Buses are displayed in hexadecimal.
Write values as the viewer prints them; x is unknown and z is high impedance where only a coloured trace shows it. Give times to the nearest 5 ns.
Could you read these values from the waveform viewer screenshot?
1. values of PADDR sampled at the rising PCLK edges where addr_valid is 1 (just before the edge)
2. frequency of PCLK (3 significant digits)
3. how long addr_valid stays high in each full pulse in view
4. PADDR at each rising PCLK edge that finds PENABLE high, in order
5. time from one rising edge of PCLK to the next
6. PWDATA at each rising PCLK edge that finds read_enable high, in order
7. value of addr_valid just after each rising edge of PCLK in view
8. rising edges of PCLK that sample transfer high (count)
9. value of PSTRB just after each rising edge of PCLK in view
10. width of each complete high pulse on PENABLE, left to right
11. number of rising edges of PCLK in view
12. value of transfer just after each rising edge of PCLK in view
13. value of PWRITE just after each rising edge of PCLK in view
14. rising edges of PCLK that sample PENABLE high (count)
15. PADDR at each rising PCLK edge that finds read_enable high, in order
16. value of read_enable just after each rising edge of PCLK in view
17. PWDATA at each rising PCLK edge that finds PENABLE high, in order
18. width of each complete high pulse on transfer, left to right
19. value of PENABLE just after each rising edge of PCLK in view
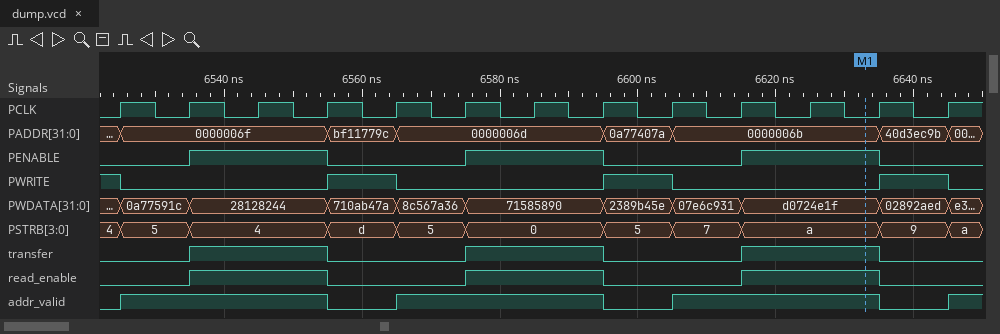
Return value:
0000006f, 0000006f, 0000006f, 0000006d, 0000006d, 0000006d, 0000006b, 0000006b, 0000006b
100 MHz
30 ns, 30 ns, 30 ns
0000006f, 0000006f, 0000006d, 0000006d, 0000006b, 0000006b
10 ns
28128244, 28128244, 71585890, 71585890, d0724e1f, d0724e1f
1 1 1 0 1 1 1 0 1 1 1 0 1
6
5, 4, 4, d, 5, 0, 0, 5, 7, a, a, 9, a
20 ns, 20 ns, 20 ns
13
0 1 1 0 0 1 1 0 0 1 1 0 0
0 0 0 1 0 0 0 1 0 0 0 1 0
6
0000006f, 0000006f, 0000006d, 0000006d, 0000006b, 0000006b
0 1 1 0 0 1 1 0 0 1 1 0 0
28128244, 28128244, 71585890, 71585890, d0724e1f, d0724e1f
20 ns, 20 ns, 20 ns
0 1 1 0 0 1 1 0 0 1 1 0 0
